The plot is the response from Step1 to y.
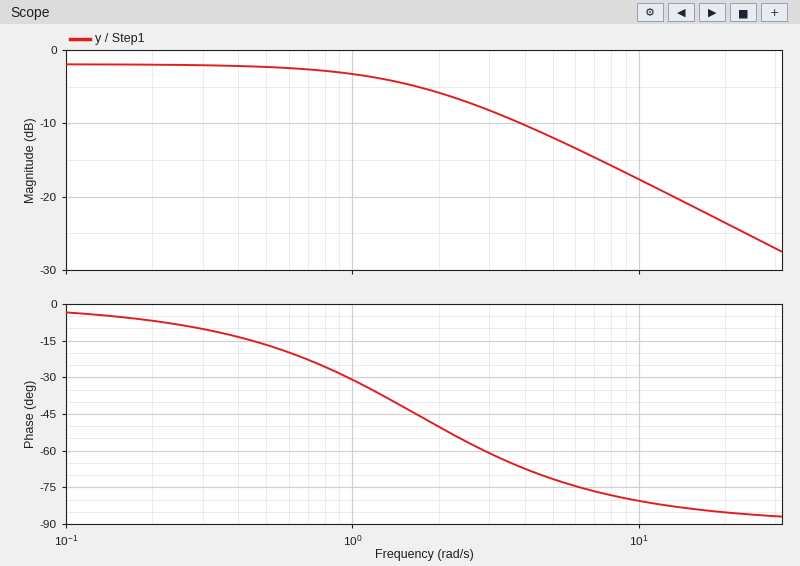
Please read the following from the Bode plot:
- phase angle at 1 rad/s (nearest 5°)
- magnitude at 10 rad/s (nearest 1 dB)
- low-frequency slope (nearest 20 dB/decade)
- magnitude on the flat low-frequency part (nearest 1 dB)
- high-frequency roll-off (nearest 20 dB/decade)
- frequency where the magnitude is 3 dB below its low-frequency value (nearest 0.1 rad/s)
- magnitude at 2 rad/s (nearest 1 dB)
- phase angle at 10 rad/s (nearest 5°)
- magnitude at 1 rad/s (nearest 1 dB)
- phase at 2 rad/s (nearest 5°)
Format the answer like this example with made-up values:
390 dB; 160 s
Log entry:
-30°; -18 dB; 0 dB/decade; -2 dB; -20 dB/decade; 1.7 rad/s; -6 dB; -80°; -3 dB; -50°
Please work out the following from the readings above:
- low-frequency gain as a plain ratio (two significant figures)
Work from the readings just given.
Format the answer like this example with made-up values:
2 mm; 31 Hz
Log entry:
0.79
